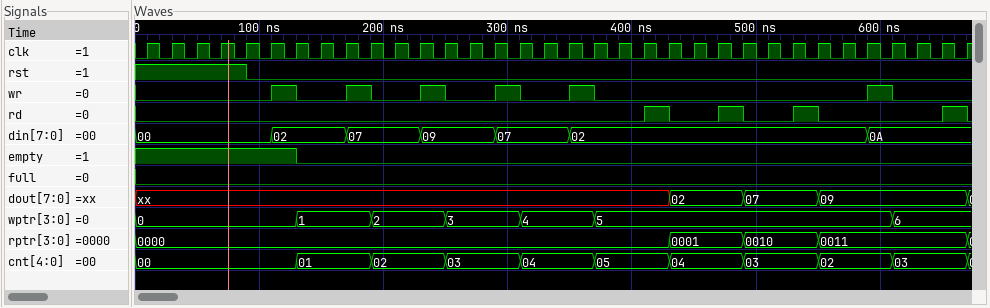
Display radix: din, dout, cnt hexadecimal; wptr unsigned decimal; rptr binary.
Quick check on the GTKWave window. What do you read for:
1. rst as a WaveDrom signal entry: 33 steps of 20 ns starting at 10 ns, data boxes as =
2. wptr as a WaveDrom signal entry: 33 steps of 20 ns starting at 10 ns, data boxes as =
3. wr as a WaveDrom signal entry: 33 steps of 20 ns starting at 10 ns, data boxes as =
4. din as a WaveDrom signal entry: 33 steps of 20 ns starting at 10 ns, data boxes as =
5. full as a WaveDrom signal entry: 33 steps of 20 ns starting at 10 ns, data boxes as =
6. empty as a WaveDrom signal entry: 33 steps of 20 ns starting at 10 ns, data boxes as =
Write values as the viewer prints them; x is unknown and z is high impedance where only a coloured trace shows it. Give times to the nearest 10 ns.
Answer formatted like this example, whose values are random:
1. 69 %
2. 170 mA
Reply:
1. {name: 'rst', wave: '1...0............................'}
2. {name: 'wptr', wave: '=.....=..=..=..=..=...........=..', data: '0 1 2 3 4 5 6'}
3. {name: 'wr', wave: '0....10.10.10.10.10..........10..'}
4. {name: 'din', wave: '=....=..=..=..=..=...........=...', data: '00 02 07 09 07 02 0A'}
5. {name: 'full', wave: '0................................'}
6. {name: 'empty', wave: '1.....0..........................'}
